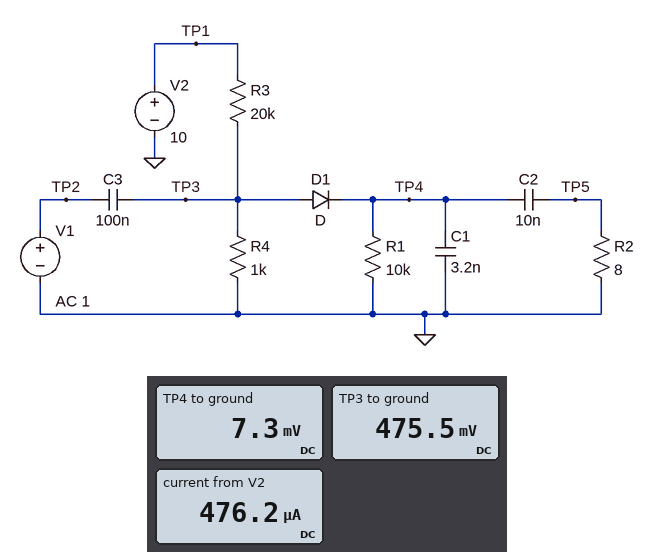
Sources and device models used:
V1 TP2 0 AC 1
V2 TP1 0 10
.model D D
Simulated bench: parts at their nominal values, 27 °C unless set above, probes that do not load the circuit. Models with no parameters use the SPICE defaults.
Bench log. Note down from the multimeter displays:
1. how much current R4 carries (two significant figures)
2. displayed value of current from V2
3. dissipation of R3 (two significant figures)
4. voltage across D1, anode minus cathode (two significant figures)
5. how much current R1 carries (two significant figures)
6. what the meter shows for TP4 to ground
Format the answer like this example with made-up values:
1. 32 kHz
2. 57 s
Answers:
1. 480 µA
2. 476.2 µA
3. 4.5 mW
4. 470 mV
5. 730 nA
6. 7.3 mV
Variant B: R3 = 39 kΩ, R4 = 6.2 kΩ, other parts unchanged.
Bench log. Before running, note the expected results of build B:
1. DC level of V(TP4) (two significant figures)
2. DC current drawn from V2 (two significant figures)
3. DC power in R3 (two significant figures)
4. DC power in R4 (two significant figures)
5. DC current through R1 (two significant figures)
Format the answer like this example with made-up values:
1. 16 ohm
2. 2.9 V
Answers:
1. 520 mV
2. 230 µA
3. 2.0 mW
4. 190 µW
5. 52 µA
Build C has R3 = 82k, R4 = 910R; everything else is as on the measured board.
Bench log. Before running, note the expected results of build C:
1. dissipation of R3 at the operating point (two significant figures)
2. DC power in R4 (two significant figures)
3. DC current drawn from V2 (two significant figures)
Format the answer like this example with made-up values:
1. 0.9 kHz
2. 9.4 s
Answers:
1. 1.2 mW
2. 13 µW
3. 120 µA
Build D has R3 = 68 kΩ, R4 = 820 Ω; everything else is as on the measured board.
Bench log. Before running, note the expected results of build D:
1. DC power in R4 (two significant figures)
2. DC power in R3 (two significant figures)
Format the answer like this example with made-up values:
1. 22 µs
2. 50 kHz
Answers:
1. 17 µW
2. 1.4 mW
